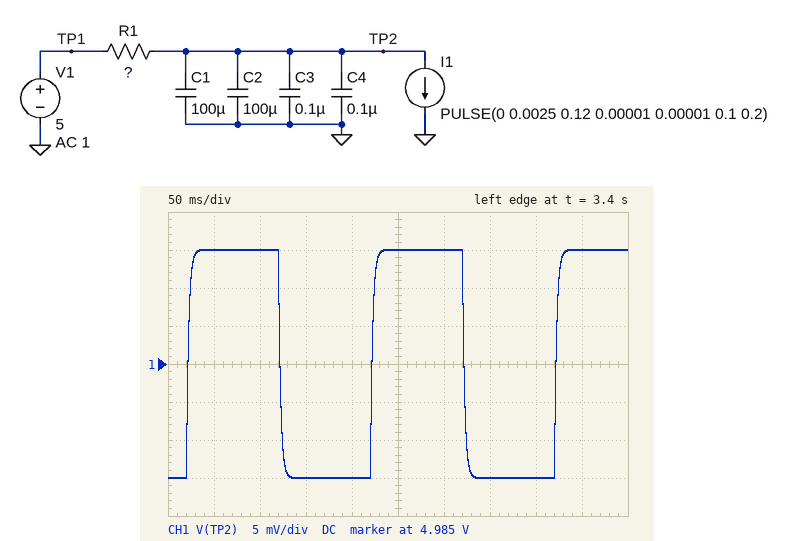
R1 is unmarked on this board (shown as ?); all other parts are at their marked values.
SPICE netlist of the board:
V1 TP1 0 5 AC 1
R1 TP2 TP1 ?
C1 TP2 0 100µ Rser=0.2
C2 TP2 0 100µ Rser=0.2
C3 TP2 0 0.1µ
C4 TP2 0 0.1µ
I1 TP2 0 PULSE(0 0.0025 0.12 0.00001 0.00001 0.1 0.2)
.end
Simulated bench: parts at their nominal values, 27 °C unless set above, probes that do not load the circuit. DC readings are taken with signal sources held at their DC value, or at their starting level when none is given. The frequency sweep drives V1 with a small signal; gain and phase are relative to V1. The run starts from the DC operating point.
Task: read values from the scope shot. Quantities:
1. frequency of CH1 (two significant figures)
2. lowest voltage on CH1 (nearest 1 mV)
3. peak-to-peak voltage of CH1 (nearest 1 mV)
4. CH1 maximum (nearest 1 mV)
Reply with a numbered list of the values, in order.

1. 5.0 Hz
2. 4.970 V
3. 30 mV
4. 5.000 V
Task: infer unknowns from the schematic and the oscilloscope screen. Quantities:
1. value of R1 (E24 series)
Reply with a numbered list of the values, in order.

1. 12 Ω
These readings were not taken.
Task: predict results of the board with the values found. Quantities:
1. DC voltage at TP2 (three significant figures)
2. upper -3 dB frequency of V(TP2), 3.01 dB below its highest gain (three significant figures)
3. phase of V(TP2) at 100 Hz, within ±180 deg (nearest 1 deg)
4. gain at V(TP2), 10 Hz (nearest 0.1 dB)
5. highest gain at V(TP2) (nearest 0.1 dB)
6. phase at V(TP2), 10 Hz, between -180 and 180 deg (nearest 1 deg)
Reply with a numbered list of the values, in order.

1. 5.00 V
2. 65.7 Hz
3. -56 deg
4. -0.1 dB
5. 0 dB
6. -9 deg
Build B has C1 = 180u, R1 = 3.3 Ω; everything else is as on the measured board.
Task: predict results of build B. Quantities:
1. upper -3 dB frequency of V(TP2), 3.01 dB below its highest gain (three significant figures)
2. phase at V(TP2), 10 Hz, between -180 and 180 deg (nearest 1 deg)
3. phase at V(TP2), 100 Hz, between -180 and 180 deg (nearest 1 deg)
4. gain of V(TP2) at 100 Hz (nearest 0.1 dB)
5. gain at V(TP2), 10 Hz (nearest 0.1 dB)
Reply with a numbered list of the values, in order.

1. 167 Hz
2. -3 deg
3. -30 deg
4. -1.3 dB
5. 0 dB
